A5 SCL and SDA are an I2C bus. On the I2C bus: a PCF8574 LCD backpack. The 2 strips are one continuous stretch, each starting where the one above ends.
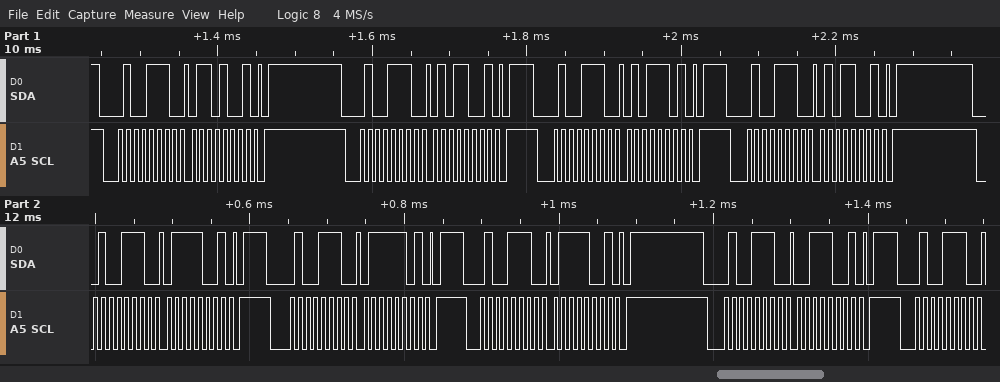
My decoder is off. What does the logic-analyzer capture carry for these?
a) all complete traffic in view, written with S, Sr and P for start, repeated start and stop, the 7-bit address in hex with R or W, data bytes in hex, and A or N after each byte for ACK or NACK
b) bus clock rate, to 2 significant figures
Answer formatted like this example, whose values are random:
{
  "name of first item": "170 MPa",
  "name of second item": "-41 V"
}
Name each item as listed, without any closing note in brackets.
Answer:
{
  "all complete traffic in view, written with S, Sr and P for start, repeated start and stop, the 7-bit address in hex with R or W, data bytes in hex, and A or N after each byte for ACK or NACK": "S 27W A 69 A P S 27W A 59 A P S 27W A 5D A P S 27W A 59 A P S 27W A 79 A P S 27W A 7D A P S 27W A 79 A P S 27W A 39 A P S 27W A",
  "bus clock rate, to 2 significant figures": "100 kHz"
}
